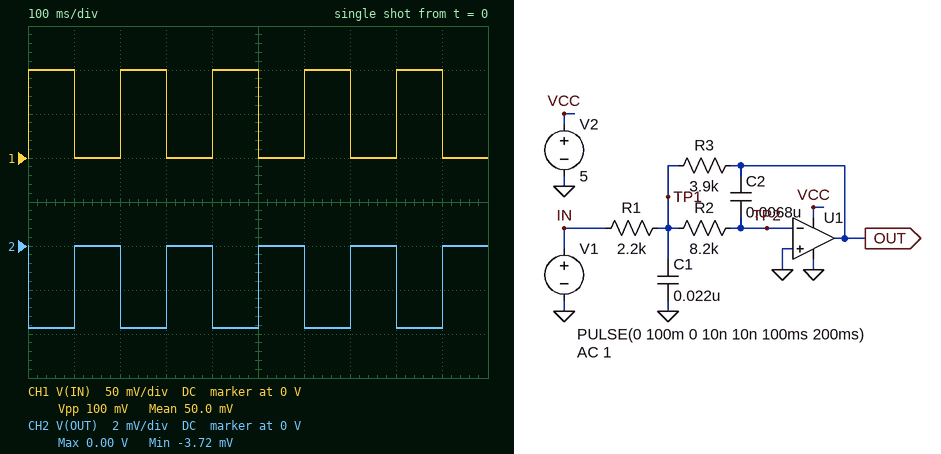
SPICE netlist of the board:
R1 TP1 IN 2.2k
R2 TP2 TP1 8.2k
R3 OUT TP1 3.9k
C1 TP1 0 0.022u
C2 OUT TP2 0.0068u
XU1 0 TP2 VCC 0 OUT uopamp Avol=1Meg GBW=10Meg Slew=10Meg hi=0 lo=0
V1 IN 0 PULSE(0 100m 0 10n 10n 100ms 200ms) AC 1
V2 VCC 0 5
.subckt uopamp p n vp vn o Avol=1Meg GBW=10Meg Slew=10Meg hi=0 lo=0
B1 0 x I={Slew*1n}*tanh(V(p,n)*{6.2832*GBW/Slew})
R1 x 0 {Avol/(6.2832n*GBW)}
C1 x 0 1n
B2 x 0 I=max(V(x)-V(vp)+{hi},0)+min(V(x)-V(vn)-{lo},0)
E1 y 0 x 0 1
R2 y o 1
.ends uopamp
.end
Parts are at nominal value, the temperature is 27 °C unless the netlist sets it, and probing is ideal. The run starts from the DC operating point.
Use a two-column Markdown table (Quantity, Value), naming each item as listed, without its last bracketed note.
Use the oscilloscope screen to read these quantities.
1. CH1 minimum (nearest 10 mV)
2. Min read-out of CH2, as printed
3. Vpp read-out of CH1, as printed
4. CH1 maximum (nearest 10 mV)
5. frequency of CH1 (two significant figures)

| Quantity | Value |
|---|---|
| CH1 minimum | 0 V |
| Min read-out of CH2, as printed | -3.72 mV |
| Vpp read-out of CH1, as printed | 100 mV |
| CH1 maximum | 100 mV |
| frequency of CH1 | 5.0 Hz |
